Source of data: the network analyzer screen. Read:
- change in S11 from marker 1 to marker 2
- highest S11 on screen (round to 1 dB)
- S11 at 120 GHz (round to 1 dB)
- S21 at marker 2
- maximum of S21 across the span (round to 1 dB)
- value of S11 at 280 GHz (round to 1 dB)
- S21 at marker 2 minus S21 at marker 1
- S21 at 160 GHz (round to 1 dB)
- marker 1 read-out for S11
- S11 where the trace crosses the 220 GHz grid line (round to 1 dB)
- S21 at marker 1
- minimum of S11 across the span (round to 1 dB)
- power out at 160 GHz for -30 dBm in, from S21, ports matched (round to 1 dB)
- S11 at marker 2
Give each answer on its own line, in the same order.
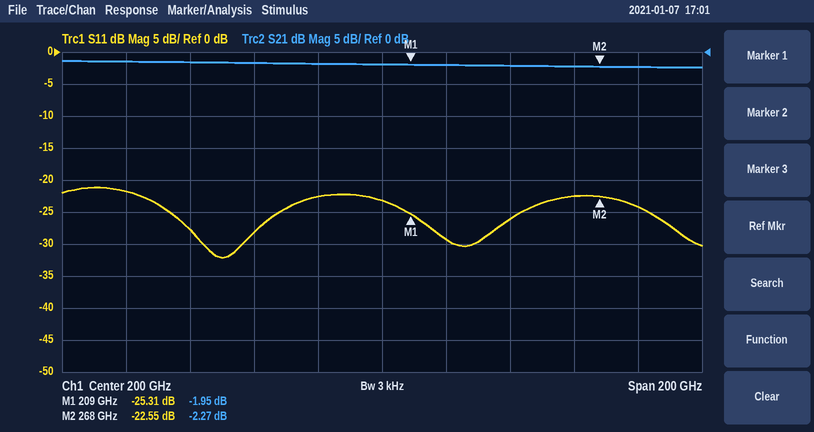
2.76 dB
-21 dB
-22 dB
-2.27 dB
-1 dB
-24 dB
-0.32 dB
-2 dB
-25.31 dB
-29 dB
-1.95 dB
-32 dB
-32 dBm
-22.55 dB
